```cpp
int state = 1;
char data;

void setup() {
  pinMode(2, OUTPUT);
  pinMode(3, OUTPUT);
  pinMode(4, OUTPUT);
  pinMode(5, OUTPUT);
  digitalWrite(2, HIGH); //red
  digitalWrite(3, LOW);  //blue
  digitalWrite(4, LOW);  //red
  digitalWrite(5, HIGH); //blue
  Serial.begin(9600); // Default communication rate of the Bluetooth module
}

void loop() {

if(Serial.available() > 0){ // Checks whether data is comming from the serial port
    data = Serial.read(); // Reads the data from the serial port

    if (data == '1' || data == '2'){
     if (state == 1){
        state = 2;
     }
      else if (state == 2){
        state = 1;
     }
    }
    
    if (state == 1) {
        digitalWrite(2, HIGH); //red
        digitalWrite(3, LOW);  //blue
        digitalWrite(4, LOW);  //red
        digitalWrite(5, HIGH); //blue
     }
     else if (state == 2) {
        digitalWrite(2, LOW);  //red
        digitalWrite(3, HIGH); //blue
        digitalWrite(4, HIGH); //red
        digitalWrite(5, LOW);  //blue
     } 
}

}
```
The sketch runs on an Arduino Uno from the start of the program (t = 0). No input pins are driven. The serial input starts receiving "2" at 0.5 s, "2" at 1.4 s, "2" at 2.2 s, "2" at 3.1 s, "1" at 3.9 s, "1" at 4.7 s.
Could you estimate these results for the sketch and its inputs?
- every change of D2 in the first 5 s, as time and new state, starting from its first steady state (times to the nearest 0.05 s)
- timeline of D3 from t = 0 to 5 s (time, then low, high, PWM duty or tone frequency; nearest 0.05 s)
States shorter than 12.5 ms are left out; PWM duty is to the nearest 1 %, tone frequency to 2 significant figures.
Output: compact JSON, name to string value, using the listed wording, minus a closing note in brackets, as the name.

{"every change of D2 in the first 5 s, as time and new state, starting from its first steady state": "0 s high; 0.5 s low; 1.4 s high; 2.2 s low; 3.1 s high; 3.9 s low; 4.7 s high", "timeline of D3 from t = 0 to 5 s": "0 s low; 0.5 s high; 1.4 s low; 2.2 s high; 3.1 s low; 3.9 s high; 4.7 s low"}
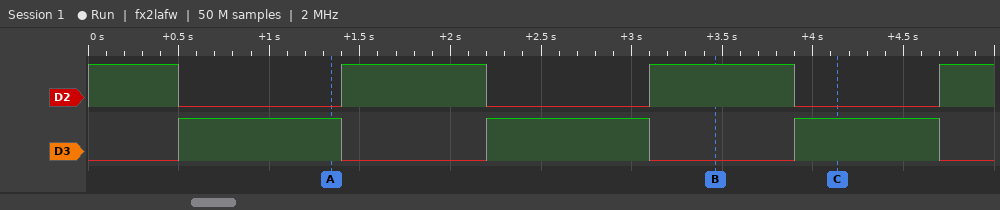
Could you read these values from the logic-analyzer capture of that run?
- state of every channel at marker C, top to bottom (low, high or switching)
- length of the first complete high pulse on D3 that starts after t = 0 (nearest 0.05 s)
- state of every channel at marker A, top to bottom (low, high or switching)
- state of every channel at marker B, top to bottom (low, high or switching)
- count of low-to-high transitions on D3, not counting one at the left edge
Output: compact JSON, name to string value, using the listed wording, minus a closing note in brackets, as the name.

{"state of every channel at marker C, top to bottom": "D2 low, D3 high", "length of the first complete high pulse on D3 that starts after t = 0": "0.90 s", "state of every channel at marker A, top to bottom": "D2 low, D3 high", "state of every channel at marker B, top to bottom": "D2 high, D3 low", "count of low-to-high transitions on D3, not counting one at the left edge": "3"}
